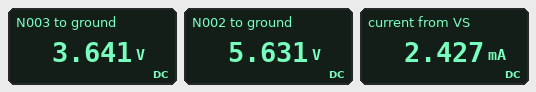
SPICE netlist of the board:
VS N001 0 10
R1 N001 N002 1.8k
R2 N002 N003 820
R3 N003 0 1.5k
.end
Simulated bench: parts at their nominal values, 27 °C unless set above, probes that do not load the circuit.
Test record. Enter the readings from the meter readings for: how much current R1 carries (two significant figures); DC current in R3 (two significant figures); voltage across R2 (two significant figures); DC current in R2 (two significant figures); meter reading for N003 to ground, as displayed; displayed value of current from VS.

2.4 mA
2.4 mA
2.0 V
2.4 mA
3.641 V
2.427 mA
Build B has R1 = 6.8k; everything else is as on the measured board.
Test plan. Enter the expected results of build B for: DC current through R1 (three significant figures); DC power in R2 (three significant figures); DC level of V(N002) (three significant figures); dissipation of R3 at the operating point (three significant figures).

1.10 mA
986 µW
2.54 V
1.80 mW
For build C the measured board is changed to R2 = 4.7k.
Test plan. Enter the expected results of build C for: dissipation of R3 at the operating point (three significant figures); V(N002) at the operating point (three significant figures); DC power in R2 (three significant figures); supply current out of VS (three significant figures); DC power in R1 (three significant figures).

2.34 mW
7.75 V
7.34 mW
1.25 mA
2.81 mW
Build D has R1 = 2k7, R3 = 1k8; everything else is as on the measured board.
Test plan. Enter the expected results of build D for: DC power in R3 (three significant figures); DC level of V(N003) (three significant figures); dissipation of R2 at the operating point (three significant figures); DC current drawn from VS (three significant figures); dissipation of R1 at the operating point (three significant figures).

6.36 mW
3.38 V
2.90 mW
1.88 mA
9.54 mW
